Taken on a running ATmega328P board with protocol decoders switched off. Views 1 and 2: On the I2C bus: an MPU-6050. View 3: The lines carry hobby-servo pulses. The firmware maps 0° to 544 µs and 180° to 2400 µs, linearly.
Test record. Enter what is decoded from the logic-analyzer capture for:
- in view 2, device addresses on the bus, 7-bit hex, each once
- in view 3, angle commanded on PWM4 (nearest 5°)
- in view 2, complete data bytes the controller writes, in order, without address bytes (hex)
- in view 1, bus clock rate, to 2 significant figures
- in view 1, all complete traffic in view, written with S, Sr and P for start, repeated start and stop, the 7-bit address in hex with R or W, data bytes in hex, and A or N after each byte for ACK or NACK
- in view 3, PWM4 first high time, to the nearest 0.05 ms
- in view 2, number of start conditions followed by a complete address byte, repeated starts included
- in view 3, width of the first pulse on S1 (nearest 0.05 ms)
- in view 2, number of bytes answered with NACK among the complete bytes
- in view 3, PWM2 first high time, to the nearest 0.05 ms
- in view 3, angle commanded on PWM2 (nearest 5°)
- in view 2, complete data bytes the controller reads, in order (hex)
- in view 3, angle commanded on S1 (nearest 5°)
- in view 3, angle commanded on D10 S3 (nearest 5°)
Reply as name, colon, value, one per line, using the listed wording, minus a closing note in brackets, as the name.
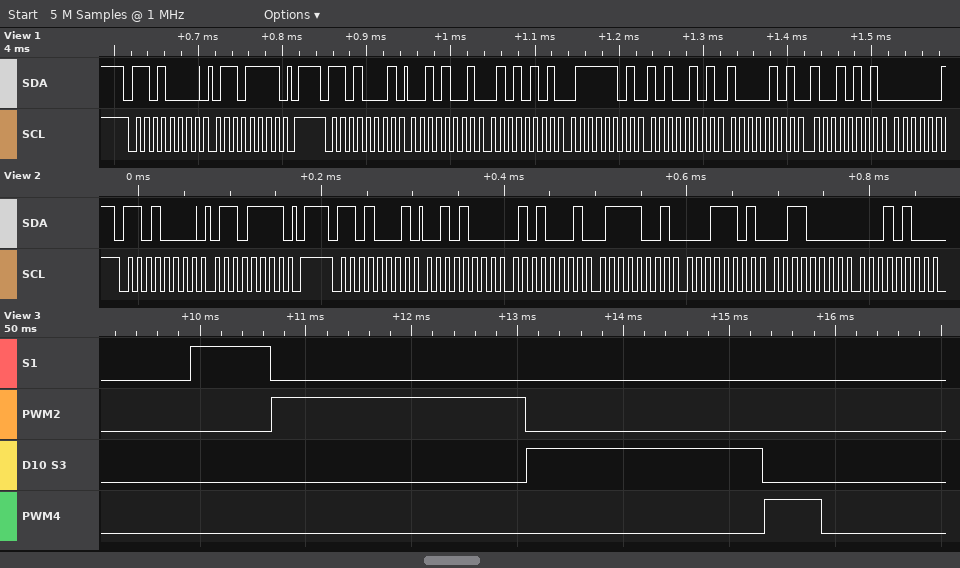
in view 2, device addresses on the bus, 7-bit hex, each once: 0x68
in view 3, angle commanded on PWM4: 0°
in view 2, complete data bytes the controller writes, in order, without address bytes: 6F
in view 1, bus clock rate, to 2 significant figures: 100 kHz
in view 1, all complete traffic in view, written with S, Sr and P for start, repeated start and stop, the 7-bit address in hex with R or W, data bytes in hex, and A or N after each byte for ACK or NACK: S 68W A 6F A P S 68R A 29 A 55 A 7D A A5 A 85 A 95 A
in view 3, PWM4 first high time, to the nearest 0.05 ms: 0.55 ms
in view 2, number of start conditions followed by a complete address byte, repeated starts included: 2
in view 3, width of the first pulse on S1: 0.75 ms
in view 2, number of bytes answered with NACK among the complete bytes: 0
in view 3, PWM2 first high time, to the nearest 0.05 ms: 2.40 ms
in view 3, angle commanded on PWM2: 180°
in view 2, complete data bytes the controller reads, in order: 28 51 79 1D 30 14
in view 3, angle commanded on S1: 20°
in view 3, angle commanded on D10 S3: 165°
